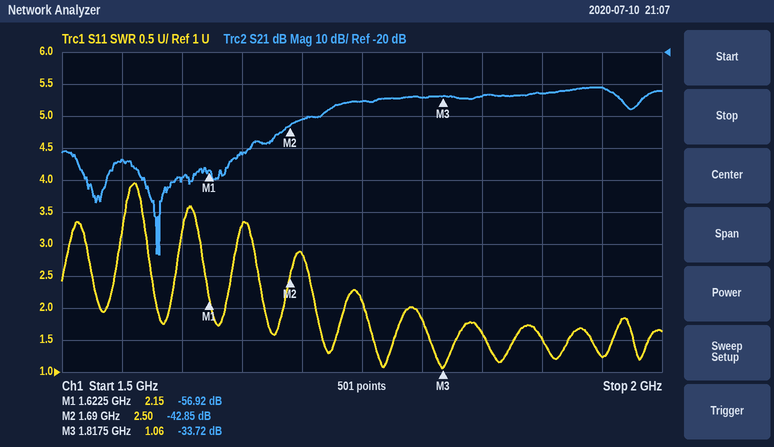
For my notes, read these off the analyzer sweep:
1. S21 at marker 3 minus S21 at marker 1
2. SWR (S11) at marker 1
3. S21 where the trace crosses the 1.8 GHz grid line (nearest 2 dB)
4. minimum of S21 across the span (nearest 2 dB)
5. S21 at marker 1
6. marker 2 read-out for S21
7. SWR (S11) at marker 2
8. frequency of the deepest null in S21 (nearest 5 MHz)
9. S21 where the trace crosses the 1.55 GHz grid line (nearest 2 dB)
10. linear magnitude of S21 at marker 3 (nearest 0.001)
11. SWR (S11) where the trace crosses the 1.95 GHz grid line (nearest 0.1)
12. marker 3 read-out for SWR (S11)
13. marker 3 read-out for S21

23.20 dB
2.15
-34 dB
-84 dB
-56.92 dB
-42.85 dB
2.50
1.580 GHz
-54 dB
0.021
1.2
1.06
-33.72 dB
